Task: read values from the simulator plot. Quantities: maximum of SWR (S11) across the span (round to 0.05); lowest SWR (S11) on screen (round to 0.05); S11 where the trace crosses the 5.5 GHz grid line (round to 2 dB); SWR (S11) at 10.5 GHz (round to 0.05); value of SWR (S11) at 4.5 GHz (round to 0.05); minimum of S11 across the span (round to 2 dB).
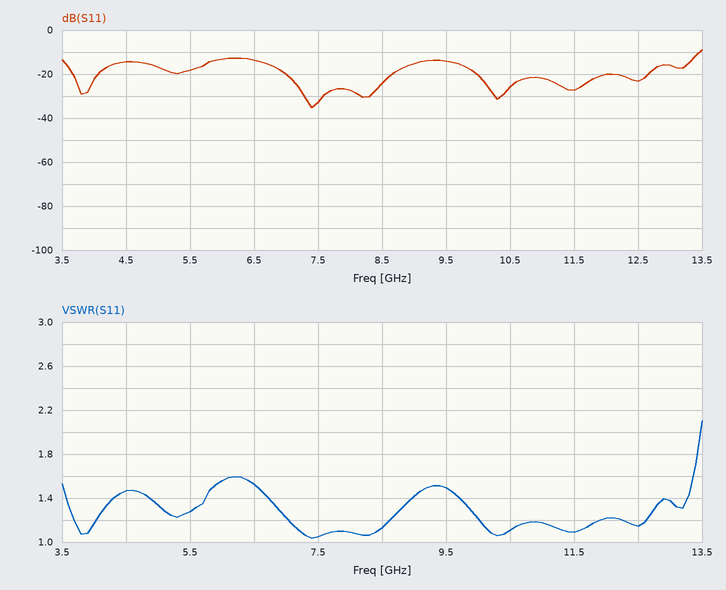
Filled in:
2.10
1.05
-18 dB
1.10
1.45
-36 dB
